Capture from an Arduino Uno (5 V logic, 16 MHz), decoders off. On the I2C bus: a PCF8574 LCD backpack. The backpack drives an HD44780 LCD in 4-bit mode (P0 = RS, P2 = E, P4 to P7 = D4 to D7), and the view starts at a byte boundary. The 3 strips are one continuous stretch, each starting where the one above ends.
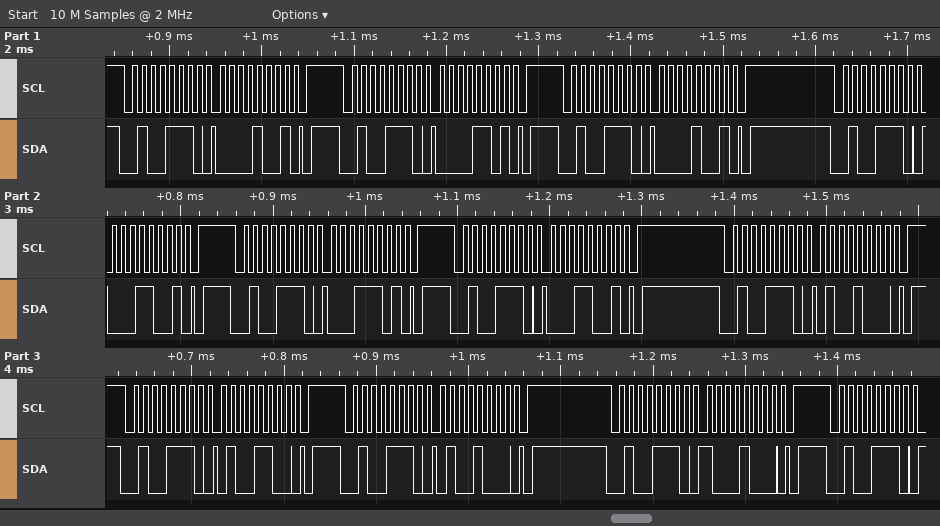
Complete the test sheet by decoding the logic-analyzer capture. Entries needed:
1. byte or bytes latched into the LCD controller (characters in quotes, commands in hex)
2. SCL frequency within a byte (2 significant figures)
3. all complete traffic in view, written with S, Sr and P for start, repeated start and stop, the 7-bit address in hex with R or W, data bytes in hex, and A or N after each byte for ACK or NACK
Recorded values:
data 0x01
100 kHz
S 27W A 09 A P S 27W A 0D A P S 27W A 09 A P S 27W A 19 A P S 27W A 1D A P S 27W A 19 A P S 27W A 48 A P S 27W A 4C A P S 27W A 48 A P S 27W A 88 A P S 27W A
